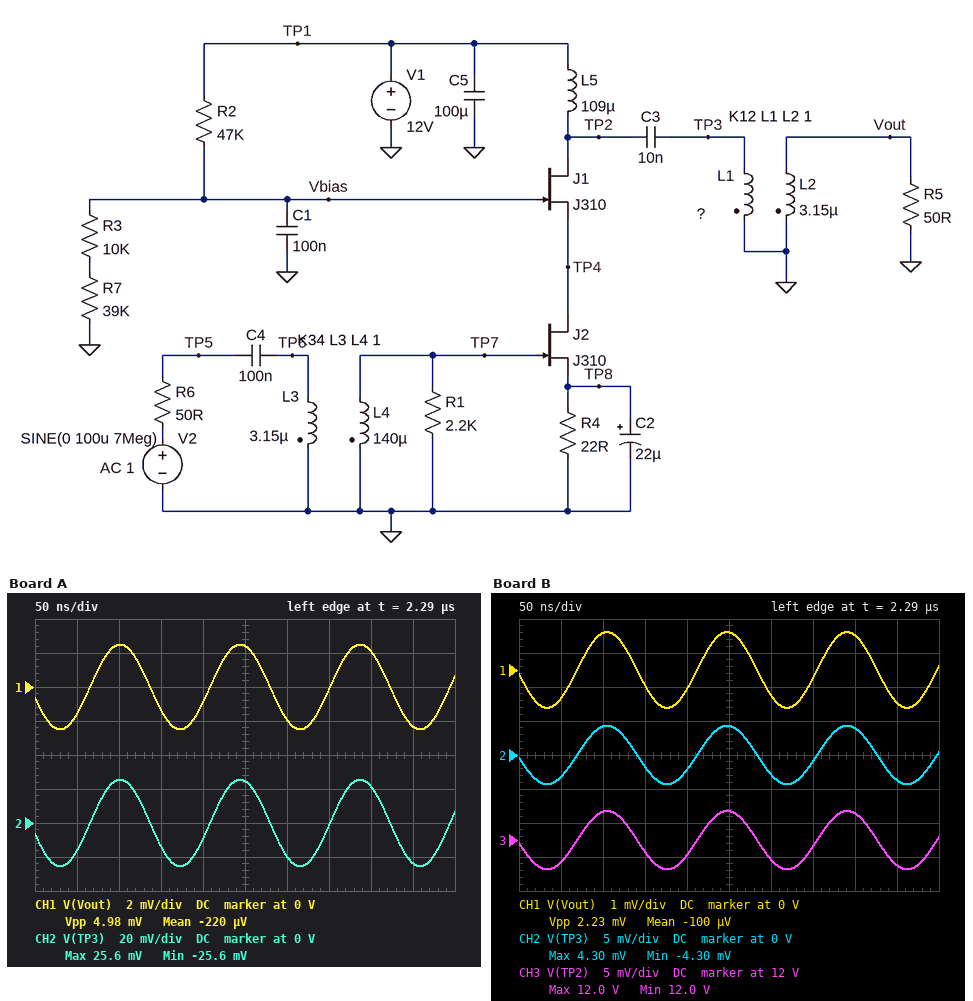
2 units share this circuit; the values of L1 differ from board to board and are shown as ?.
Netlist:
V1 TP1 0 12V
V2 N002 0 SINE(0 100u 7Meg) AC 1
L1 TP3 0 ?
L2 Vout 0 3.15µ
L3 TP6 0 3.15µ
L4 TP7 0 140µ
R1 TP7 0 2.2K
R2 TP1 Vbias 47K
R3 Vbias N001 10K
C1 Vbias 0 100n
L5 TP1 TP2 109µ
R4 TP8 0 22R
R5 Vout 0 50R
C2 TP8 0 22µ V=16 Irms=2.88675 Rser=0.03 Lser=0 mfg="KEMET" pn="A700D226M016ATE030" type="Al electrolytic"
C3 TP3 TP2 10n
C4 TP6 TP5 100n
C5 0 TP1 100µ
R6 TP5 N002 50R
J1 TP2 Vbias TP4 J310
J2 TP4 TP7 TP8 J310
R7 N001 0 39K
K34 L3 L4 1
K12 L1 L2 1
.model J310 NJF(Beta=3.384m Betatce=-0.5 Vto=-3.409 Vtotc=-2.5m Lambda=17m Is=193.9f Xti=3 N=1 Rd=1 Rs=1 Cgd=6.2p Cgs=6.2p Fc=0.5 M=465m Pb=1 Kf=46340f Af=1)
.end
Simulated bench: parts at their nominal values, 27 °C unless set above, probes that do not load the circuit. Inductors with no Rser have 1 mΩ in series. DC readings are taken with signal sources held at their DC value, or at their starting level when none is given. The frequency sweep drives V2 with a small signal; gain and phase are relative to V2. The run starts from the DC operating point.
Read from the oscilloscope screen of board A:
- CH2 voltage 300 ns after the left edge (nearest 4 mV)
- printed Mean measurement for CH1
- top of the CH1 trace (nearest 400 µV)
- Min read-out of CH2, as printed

-20 mV
-220 µV
2.4 mV
-25.6 mV
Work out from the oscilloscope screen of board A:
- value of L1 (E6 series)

330 µH
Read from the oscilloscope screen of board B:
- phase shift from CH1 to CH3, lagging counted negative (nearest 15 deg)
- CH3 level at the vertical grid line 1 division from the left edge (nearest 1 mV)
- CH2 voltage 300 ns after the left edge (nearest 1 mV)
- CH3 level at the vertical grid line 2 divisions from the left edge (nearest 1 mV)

0 deg
11.997 V
-3 mV
12.004 V
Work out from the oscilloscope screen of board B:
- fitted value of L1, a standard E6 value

47 µH
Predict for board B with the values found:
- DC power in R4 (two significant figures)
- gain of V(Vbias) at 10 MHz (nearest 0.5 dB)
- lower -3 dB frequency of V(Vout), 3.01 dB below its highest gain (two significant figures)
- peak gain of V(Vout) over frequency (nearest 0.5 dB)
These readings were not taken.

18 mW
-59.0 dB
2.9 MHz
21.0 dB
